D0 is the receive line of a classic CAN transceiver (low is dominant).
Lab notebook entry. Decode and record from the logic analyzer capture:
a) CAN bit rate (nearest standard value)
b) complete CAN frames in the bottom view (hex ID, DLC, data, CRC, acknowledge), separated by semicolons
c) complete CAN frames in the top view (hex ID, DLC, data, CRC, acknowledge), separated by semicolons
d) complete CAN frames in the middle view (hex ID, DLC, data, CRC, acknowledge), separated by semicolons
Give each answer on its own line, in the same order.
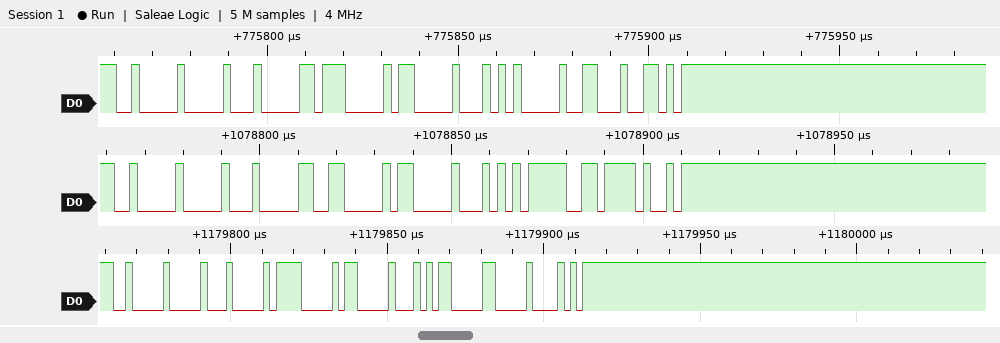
500 kbit/s
ID 200, DLC 4, data 0F 03 00 AC, CRC 0802, ACK
ID 200, DLC 4, data 17 03 00 A8, CRC 0626, ACK
ID 200, DLC 4, data 13 03 00 AB, CRC 76F4, ACK
